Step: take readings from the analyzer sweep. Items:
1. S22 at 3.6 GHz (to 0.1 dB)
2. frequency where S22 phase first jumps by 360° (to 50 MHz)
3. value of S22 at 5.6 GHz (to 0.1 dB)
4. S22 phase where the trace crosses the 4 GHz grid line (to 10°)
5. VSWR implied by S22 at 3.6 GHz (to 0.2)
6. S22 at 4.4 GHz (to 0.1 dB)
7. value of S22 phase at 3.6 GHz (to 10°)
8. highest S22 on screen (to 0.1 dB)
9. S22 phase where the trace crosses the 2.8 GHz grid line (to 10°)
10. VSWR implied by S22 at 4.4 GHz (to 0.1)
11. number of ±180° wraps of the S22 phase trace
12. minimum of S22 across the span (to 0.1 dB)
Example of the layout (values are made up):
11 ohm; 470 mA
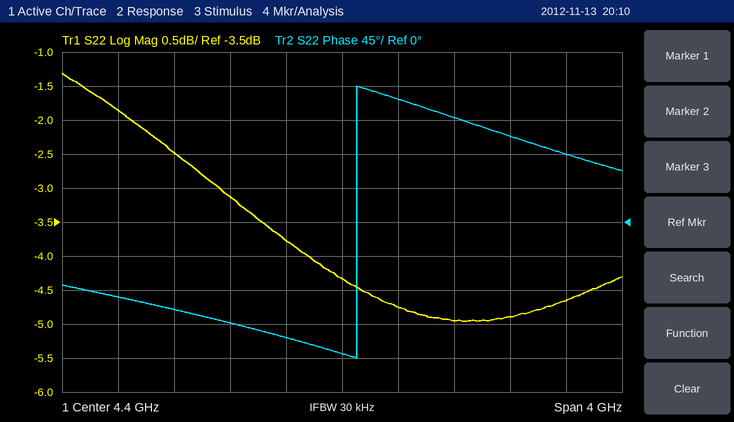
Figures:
-3.1 dB; 4.50 GHz; -4.9 dB; -150°; 5.6; -4.3 dB; -130°; -1.3 dB; -100°; 4.1; 1; -5.0 dB
